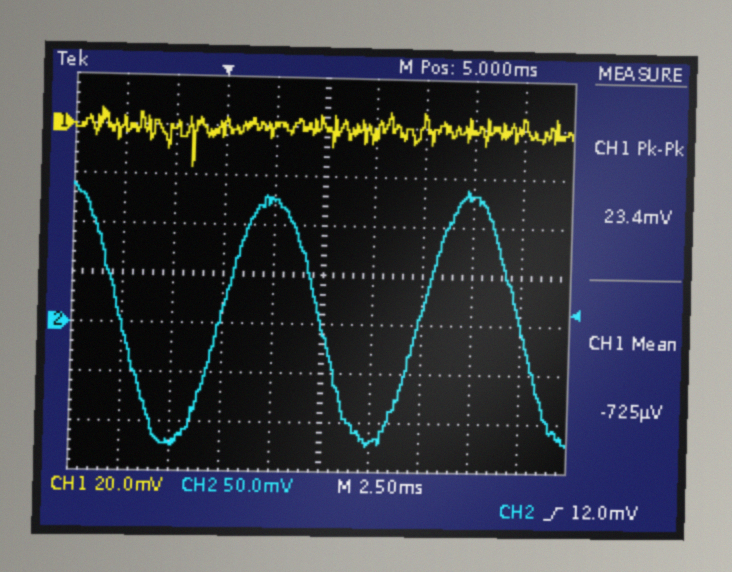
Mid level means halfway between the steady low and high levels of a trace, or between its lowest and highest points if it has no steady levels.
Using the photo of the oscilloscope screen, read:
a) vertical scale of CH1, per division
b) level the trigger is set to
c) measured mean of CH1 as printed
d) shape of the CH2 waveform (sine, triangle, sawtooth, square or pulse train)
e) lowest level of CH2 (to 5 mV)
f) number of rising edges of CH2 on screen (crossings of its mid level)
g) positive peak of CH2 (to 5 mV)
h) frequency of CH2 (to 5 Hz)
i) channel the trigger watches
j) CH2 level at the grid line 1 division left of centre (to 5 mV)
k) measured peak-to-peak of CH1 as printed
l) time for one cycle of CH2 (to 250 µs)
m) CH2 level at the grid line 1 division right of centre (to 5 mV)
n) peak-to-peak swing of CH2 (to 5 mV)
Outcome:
20 mV
12.0 mV
-725 µV
sine
-125 mV
2
140 mV
100 Hz
CH2
125 mV
23.4 mV
10.00 ms
-120 mV
265 mV
